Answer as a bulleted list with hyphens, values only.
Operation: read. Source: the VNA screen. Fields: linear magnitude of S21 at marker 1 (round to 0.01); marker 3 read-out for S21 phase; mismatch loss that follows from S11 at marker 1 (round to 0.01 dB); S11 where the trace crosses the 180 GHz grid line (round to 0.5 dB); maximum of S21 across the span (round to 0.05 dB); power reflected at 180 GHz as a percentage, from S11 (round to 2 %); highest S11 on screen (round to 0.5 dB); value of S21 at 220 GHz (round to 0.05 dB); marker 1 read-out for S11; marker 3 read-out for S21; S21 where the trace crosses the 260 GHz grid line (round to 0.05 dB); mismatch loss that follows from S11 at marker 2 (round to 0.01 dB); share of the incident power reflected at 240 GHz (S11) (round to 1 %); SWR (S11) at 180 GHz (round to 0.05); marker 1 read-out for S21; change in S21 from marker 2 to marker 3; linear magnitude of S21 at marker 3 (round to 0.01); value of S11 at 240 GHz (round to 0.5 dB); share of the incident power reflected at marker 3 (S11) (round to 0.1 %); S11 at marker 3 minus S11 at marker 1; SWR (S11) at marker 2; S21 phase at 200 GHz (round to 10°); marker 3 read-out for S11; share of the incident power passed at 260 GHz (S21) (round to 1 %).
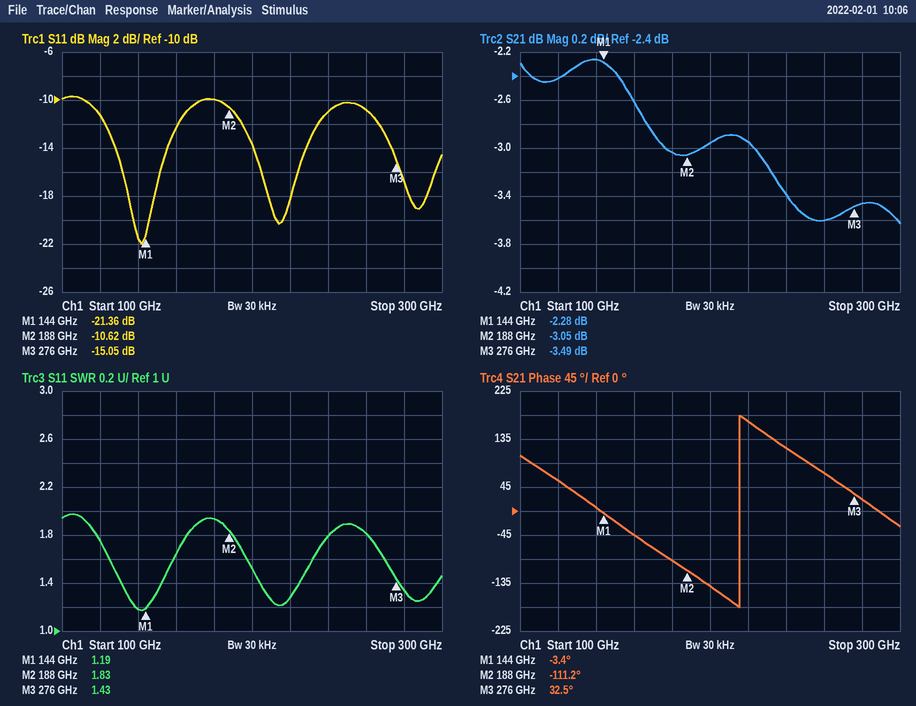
- 0.77
- 32.5°
- 0.03 dB
- -10.0 dB
- -2.25 dB
- 10 %
- -9.5 dB
- -2.95 dB
- -21.36 dB
- -3.49 dB
- -3.60 dB
- 0.39 dB
- 8 %
- 1.95
- -2.28 dB
- -0.44 dB
- 0.67
- -11.0 dB
- 3.1 %
- 6.31 dB
- 1.83
- -140°
- -15.05 dB
- 44 %
